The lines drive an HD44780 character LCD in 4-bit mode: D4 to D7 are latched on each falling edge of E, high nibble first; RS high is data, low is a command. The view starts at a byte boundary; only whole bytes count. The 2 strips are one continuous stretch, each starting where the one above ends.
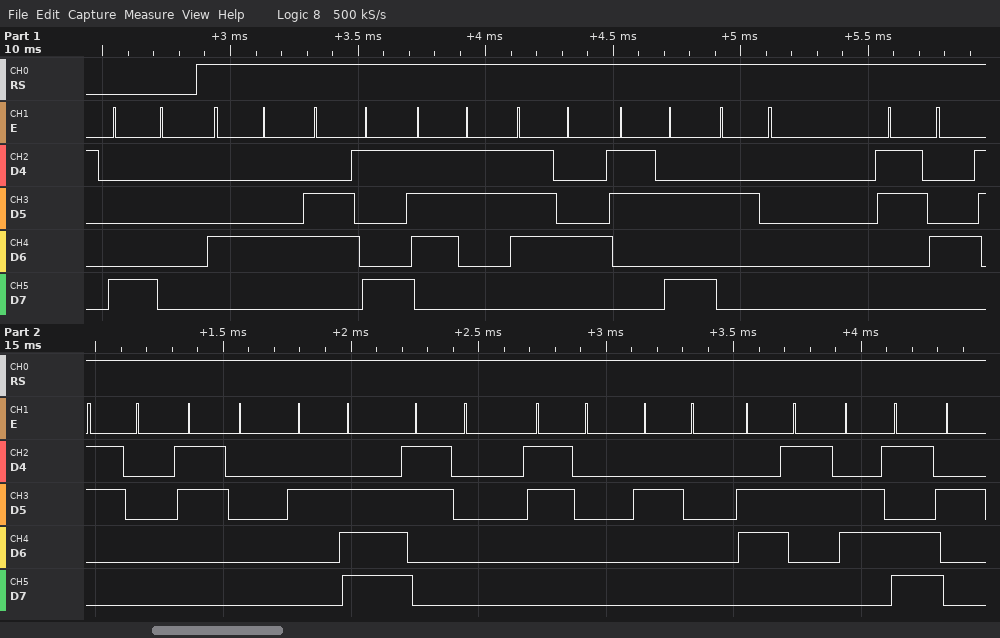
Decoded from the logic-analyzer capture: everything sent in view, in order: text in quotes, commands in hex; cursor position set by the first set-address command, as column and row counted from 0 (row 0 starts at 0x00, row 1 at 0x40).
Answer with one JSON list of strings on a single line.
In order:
["0x80 \"Dist: 400.00 cm\"", "column 0, row 0"]
